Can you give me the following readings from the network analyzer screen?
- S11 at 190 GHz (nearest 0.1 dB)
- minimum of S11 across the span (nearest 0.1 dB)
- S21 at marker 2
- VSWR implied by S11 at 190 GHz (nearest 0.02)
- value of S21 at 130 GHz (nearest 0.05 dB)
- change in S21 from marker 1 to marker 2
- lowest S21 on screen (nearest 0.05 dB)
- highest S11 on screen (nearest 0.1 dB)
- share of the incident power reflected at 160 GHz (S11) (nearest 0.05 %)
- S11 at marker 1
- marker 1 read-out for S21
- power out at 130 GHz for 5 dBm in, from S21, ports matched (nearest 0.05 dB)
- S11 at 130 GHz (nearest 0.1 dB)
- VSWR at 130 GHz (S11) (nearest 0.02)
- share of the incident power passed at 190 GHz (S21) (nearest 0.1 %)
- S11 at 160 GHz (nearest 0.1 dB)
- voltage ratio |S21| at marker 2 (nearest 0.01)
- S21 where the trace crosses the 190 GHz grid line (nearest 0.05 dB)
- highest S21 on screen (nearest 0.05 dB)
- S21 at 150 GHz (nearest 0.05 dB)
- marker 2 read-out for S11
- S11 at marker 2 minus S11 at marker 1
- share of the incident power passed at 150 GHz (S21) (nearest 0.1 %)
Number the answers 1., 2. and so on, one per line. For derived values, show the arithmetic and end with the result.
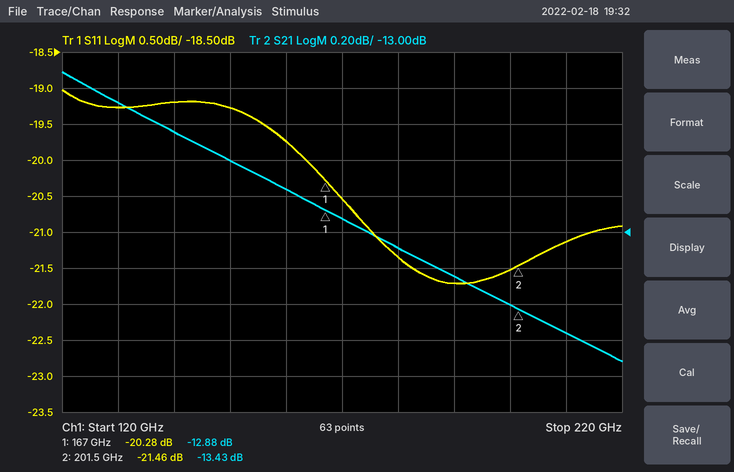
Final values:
1. -21.7 dB
2. -21.7 dB
3. -13.43 dB
4. |Γ| = 10^(-21.7/20) = 0.0822; VSWR = (1 + 0.0822)/(1 − 0.0822) ≈ 1.18
5. -12.30 dB
6. -13.43 − (-12.88) = -0.55 dB
7. -13.70 dB
8. -19.0 dB
9. 10^(-19.7/10) ≈ 1.07 %, so 1.05 % to the nearest 0.05 %
10. -20.28 dB
11. -12.88 dB
12. 5 dBm + (-12.30 dB) = -7.30 dBm
13. -19.3 dB
14. |Γ| = 10^(-19.3/20) = 0.1084; VSWR = (1 + 0.1084)/(1 − 0.1084) ≈ 1.24
15. 10^(-13.25/10) ≈ 4.7 %
16. -19.7 dB
17. 10^(-13.43/20) ≈ 0.21
18. -13.25 dB
19. -12.10 dB
20. -12.60 dB
21. -21.46 dB
22. -21.46 − (-20.28) = -1.18 dB
23. 10^(-12.6/10) ≈ 5.5 %
